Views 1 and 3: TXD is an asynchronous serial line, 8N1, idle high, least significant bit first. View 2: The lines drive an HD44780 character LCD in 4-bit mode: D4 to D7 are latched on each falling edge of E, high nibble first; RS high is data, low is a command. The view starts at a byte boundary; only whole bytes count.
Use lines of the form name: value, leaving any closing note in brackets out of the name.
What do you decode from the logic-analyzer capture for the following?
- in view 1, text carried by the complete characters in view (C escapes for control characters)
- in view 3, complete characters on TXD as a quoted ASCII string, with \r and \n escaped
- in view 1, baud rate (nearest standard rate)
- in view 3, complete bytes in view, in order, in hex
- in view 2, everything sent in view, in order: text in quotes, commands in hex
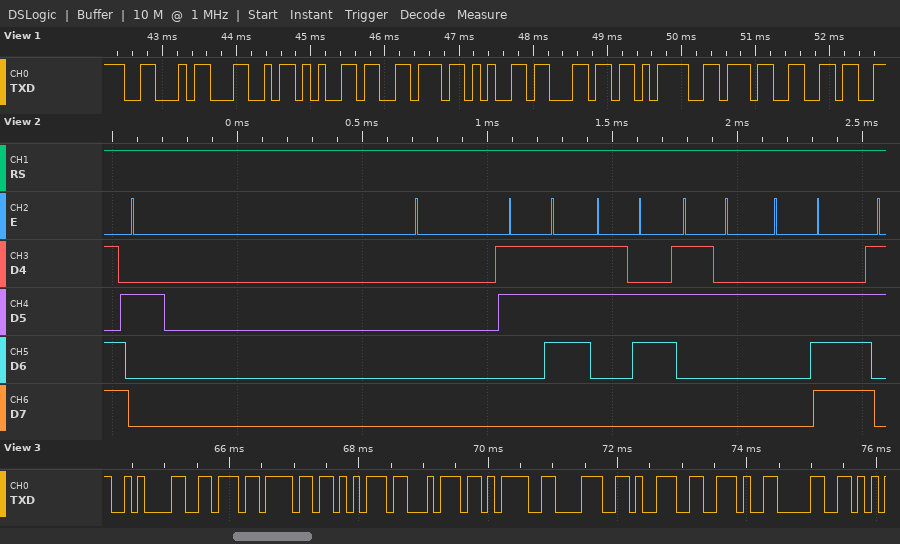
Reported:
in view 1, text carried by the complete characters in view: "FLevel=76"
in view 3, complete characters on TXD as a quoted ASCII string, with \r and \n escaped: "\nvout=89.0"
in view 1, baud rate: 9600 baud
in view 3, complete bytes in view, in order, in hex: 0x0A 0x76 0x6F 0x75 0x74 0x3D 0x38 0x39 0x2E 0x30
in view 2, everything sent in view, in order: text in quotes, commands in hex: " 762."
